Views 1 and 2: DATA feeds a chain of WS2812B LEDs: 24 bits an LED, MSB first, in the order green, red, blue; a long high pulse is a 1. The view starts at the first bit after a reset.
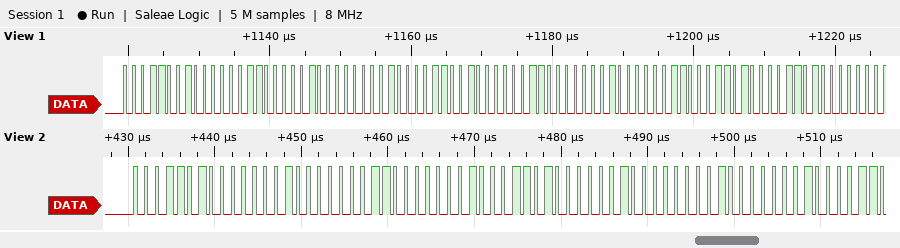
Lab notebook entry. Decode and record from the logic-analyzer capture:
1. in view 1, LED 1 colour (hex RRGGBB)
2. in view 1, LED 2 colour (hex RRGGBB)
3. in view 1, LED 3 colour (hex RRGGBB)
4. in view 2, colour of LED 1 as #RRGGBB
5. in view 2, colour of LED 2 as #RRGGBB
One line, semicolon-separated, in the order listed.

#031904; #190203; #03011A; #021A03; #1A0104
